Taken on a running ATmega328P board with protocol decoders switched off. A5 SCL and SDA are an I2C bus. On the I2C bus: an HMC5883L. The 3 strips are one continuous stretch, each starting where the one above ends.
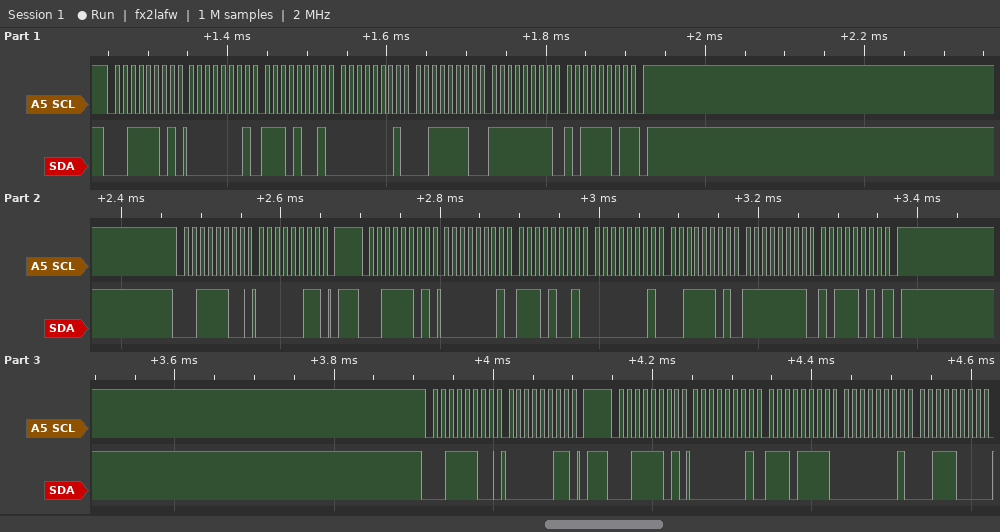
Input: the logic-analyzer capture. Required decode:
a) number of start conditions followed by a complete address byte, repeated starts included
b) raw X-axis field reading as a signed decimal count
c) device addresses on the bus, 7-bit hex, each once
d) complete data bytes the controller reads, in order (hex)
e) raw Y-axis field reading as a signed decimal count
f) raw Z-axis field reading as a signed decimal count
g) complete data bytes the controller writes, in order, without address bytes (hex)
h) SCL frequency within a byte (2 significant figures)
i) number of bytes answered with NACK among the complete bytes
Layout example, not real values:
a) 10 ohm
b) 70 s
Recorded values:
a) 5
b) 489
c) 0x1E
d) 01 E9 01 3E FF BD 01 E9 01 3D FF BA 01 EF 01 38
e) -70
f) 317
g) 03 03
h) 100 kHz
i) 2
